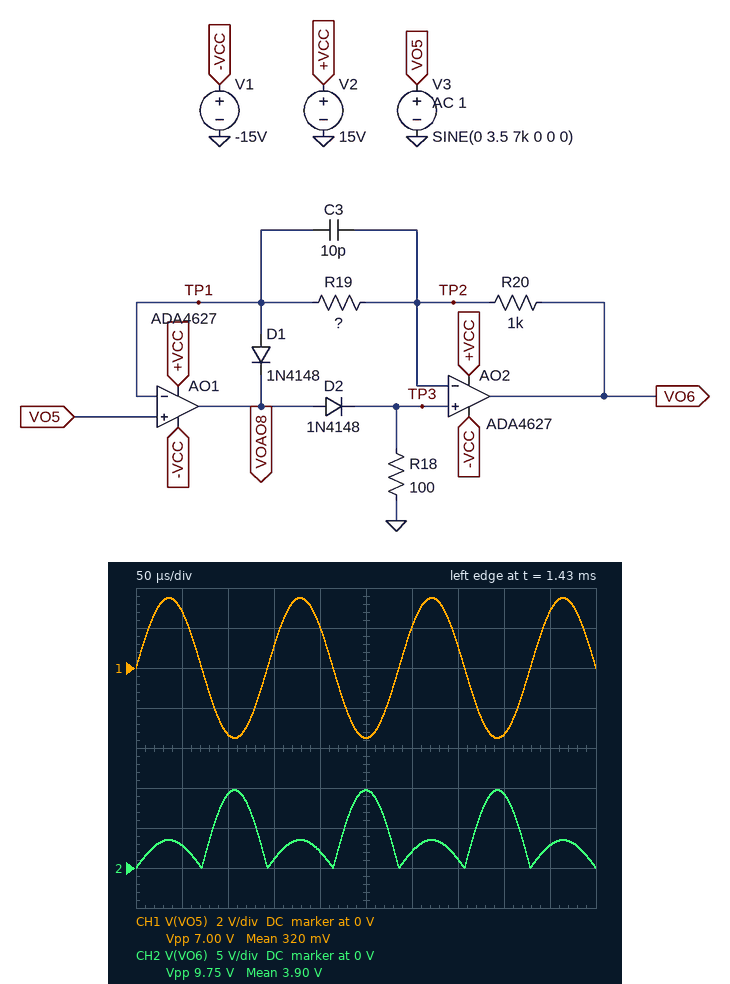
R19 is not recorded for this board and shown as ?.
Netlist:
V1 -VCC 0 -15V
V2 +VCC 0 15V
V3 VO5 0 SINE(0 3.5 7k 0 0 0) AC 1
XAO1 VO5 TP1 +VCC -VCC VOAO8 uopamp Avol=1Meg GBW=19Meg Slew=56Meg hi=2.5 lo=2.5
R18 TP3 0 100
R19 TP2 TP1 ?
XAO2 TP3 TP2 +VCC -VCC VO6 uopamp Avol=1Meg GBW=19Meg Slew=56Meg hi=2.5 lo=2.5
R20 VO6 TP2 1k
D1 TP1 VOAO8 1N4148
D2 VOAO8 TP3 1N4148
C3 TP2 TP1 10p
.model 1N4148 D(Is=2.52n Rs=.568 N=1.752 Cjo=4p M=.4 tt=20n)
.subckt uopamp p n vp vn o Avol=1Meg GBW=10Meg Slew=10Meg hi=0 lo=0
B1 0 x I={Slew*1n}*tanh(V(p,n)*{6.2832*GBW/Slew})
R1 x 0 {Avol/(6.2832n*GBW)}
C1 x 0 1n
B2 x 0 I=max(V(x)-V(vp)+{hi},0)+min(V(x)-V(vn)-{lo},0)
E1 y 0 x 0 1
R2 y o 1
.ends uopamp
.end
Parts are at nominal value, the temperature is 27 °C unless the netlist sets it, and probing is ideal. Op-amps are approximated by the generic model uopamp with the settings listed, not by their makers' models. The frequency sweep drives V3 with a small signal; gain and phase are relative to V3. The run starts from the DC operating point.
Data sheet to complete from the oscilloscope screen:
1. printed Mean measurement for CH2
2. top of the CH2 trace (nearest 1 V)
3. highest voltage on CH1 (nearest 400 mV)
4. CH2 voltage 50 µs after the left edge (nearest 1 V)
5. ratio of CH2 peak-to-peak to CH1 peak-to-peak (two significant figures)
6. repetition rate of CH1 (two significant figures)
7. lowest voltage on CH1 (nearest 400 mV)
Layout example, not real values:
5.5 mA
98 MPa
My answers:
3.90 V
10 V
3.6 V
3 V
1.4
7.0 kHz
-3.6 V
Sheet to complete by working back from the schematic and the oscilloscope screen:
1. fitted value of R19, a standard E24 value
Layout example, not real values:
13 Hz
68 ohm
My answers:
360 Ω
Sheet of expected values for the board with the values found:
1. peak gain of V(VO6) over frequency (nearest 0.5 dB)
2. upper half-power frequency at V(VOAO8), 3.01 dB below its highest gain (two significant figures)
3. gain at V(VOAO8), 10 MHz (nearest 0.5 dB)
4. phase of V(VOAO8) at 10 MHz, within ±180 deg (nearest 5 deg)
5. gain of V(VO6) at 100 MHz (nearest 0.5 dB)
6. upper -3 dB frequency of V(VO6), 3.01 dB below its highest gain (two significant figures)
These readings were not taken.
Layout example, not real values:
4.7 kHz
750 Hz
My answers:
5.5 dB
410 Hz
3.0 dB
-95 deg
-32.0 dB
430 Hz
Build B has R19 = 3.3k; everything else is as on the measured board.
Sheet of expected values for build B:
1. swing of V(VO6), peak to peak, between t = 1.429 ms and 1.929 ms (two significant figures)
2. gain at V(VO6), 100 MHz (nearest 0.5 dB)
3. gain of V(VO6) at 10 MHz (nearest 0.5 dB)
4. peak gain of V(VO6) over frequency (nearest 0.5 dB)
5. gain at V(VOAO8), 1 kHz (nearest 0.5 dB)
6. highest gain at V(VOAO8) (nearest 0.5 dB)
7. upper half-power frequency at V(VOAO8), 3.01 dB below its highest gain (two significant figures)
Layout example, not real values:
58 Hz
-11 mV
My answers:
3.5 V
-31.5 dB
-13.0 dB
-11.5 dB
72.5 dB
74.5 dB
1.4 kHz
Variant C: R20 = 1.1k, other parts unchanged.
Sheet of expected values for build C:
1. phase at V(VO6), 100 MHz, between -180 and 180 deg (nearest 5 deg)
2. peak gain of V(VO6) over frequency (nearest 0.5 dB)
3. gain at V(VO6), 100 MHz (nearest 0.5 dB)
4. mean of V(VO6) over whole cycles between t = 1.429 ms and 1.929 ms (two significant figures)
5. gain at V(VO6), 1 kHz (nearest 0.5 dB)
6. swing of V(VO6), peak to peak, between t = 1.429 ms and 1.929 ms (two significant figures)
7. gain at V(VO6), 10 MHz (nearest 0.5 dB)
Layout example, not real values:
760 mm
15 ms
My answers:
20 deg
6.5 dB
-31.5 dB
4.5 V
-1.0 dB
11 V
-9.5 dB
